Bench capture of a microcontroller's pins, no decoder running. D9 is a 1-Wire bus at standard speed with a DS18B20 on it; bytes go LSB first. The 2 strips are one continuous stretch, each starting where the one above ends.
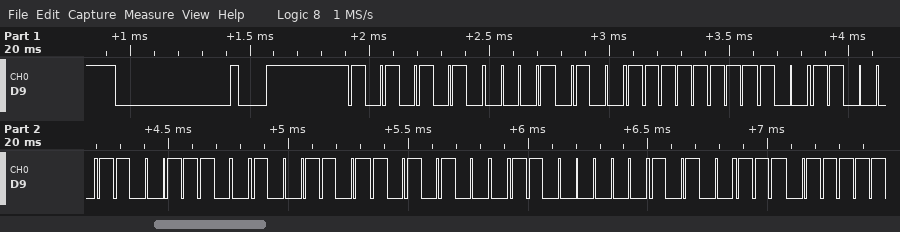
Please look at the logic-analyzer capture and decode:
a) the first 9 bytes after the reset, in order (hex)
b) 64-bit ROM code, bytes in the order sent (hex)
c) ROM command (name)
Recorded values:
55 28 FF 19 73 B2 15 03 E5
28 FF 19 73 B2 15 03 E5
Match ROM
